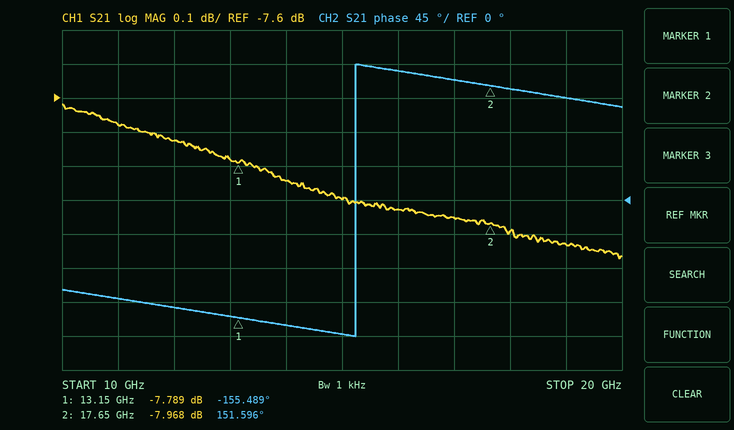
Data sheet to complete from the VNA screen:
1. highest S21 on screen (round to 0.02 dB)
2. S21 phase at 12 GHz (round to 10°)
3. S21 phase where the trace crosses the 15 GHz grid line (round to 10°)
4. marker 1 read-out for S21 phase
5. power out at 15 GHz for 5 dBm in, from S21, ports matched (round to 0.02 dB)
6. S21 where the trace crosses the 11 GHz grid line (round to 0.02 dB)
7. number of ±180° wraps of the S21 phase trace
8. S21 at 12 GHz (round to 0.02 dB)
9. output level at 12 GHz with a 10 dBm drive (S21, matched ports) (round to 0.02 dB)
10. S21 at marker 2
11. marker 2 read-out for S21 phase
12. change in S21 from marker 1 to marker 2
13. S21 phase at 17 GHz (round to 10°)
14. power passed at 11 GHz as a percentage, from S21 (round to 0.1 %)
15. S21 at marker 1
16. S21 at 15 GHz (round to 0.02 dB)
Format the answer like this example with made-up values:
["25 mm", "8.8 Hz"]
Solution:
["-7.62 dB", "-140°", "-180°", "-155.489°", "-2.90 dBm", "-7.68 dB", "1", "-7.72 dB", "2.28 dBm", "-7.968 dB", "151.596°", "-0.179 dB", "160°", "17.1 %", "-7.789 dB", "-7.90 dB"]
